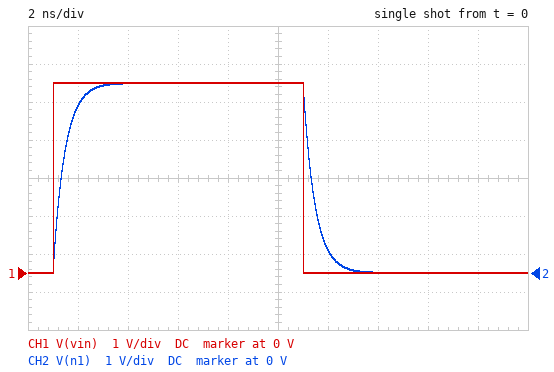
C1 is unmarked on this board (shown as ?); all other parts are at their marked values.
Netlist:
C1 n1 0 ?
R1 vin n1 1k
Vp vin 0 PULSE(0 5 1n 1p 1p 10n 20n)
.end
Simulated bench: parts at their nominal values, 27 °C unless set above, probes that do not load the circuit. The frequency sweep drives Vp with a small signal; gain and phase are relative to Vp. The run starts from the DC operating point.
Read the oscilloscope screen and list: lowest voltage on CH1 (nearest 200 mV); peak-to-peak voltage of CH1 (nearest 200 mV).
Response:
0 V
5.0 V
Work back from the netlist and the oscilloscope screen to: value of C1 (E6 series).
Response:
470 fF
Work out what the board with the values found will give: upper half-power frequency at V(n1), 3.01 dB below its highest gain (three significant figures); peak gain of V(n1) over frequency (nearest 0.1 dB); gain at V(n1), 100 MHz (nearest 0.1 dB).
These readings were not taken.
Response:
339 MHz
0 dB
-0.4 dB
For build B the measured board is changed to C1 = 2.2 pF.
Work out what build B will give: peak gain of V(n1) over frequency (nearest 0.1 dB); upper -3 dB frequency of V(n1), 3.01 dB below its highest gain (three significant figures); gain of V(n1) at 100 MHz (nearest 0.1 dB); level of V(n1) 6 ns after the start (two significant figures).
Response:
0 dB
72.3 MHz
-4.6 dB
4.5 V
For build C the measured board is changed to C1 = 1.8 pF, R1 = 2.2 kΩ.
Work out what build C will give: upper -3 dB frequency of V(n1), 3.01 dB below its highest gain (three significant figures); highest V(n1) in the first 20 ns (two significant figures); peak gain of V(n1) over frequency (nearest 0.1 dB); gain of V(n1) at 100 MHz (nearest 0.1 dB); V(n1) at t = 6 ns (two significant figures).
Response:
40.2 MHz
4.6 V
0 dB
-8.6 dB
3.6 V
